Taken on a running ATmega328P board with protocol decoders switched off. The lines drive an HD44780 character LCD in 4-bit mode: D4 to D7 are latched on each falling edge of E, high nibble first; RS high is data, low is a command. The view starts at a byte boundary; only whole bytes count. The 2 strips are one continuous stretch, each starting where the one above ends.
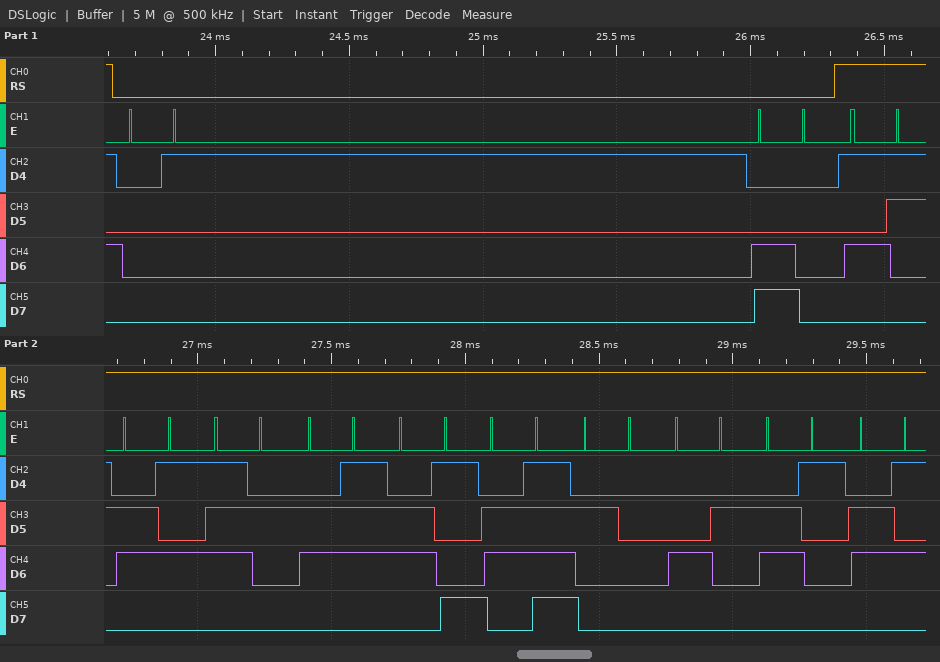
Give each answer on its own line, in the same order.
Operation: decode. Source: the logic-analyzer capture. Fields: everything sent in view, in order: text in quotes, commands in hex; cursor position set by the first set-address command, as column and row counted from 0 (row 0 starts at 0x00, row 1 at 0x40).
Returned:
0x01 0xC0 "Sergio Bae"
column 0, row 1
